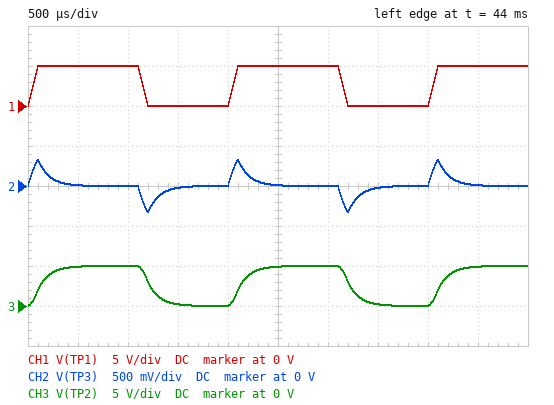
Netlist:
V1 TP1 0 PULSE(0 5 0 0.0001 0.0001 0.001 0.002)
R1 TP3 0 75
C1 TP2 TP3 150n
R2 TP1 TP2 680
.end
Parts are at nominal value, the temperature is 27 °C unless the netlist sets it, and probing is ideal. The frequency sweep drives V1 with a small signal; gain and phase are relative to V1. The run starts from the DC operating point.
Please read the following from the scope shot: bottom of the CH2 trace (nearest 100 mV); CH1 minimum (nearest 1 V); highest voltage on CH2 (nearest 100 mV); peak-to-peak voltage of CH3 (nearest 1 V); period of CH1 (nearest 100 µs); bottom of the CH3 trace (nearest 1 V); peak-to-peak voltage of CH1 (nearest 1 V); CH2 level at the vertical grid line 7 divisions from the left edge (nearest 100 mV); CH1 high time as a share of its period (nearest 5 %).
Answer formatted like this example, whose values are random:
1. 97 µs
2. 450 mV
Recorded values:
1. -300 mV
2. 0 V
3. 300 mV
4. 5 V
5. 2.0 ms
6. 0 V
7. 5 V
8. 0 V
9. 55 %
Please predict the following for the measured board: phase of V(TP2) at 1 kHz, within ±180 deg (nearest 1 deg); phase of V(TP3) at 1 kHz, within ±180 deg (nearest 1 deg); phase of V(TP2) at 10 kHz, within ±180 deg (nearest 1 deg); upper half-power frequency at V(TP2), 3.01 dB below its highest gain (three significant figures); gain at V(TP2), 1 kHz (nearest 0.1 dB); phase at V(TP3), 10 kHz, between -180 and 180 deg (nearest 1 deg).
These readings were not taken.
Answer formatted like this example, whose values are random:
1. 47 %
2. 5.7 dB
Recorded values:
1. -31 deg
2. 55 deg
3. -47 deg
4. 1.42 kHz
5. -1.8 dB
6. 8 deg
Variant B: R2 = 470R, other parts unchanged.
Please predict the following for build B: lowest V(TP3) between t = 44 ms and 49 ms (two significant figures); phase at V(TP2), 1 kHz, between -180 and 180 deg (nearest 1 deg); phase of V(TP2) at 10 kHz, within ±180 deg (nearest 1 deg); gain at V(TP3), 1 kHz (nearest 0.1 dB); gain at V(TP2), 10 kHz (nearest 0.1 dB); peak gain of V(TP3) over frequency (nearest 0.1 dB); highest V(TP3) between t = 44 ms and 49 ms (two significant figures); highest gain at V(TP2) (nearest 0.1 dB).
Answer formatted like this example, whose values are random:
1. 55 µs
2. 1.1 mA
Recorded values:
1. -400 mV
2. -23 deg
3. -44 deg
4. -24.0 dB
5. -12.6 dB
6. -17.2 dB
7. 400 mV
8. 0 dB
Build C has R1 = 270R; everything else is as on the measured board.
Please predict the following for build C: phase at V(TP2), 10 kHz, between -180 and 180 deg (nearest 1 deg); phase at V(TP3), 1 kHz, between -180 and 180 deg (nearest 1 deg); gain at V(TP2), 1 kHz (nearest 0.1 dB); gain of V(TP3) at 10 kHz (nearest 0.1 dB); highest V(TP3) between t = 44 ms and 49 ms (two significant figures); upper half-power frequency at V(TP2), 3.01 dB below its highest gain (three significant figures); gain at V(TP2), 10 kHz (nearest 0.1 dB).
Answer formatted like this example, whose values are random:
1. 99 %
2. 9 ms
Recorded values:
1. -15 deg
2. 48 deg
3. -2.3 dB
4. -11.0 dB
5. 1.0 V
6. 1.22 kHz
7. -10.4 dB
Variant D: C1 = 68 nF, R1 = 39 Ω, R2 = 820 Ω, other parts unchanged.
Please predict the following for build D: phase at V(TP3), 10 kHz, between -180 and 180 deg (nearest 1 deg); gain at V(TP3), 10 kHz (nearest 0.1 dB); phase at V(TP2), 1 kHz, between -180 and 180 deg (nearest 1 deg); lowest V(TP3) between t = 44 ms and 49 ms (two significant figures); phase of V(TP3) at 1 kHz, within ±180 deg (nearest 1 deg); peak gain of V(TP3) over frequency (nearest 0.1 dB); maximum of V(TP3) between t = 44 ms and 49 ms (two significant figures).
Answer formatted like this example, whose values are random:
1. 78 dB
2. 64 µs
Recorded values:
1. 15 deg
2. -27.2 dB
3. -19 deg
4. -110 mV
5. 70 deg
6. -26.9 dB
7. 110 mV
